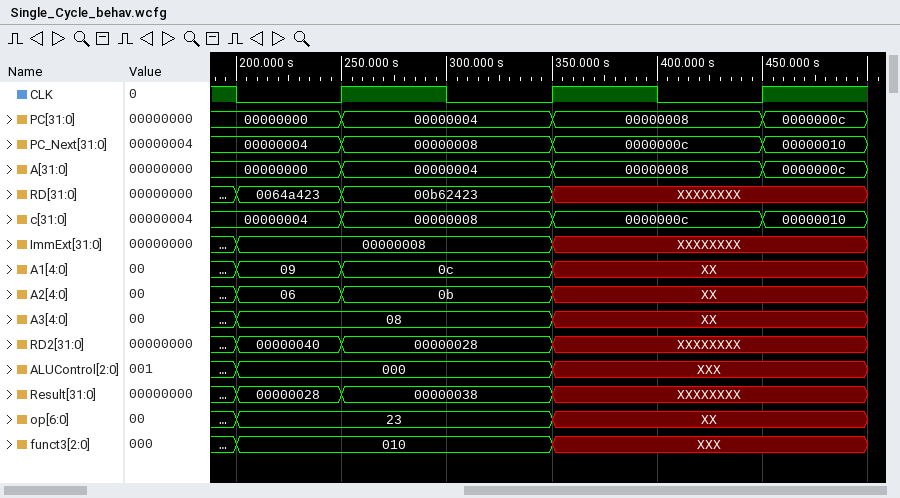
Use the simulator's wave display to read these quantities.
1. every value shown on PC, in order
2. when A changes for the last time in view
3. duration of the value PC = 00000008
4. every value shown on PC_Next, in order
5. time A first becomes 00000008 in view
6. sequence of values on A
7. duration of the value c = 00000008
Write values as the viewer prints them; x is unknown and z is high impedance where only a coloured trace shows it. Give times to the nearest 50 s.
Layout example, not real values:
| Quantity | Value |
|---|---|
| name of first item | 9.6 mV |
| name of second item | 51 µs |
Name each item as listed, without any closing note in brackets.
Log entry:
| Quantity | Value |
|---|---|
| every value shown on PC, in order | 00000000, 00000004, 00000008, 0000000c |
| when A changes for the last time in view | 450 s |
| duration of the value PC = 00000008 | 100 s |
| every value shown on PC_Next, in order | 00000004, 00000008, 0000000c, 00000010 |
| time A first becomes 00000008 in view | 350 s |
| sequence of values on A | 00000000, 00000004, 00000008, 0000000c |
| duration of the value c = 00000008 | 100 s |
